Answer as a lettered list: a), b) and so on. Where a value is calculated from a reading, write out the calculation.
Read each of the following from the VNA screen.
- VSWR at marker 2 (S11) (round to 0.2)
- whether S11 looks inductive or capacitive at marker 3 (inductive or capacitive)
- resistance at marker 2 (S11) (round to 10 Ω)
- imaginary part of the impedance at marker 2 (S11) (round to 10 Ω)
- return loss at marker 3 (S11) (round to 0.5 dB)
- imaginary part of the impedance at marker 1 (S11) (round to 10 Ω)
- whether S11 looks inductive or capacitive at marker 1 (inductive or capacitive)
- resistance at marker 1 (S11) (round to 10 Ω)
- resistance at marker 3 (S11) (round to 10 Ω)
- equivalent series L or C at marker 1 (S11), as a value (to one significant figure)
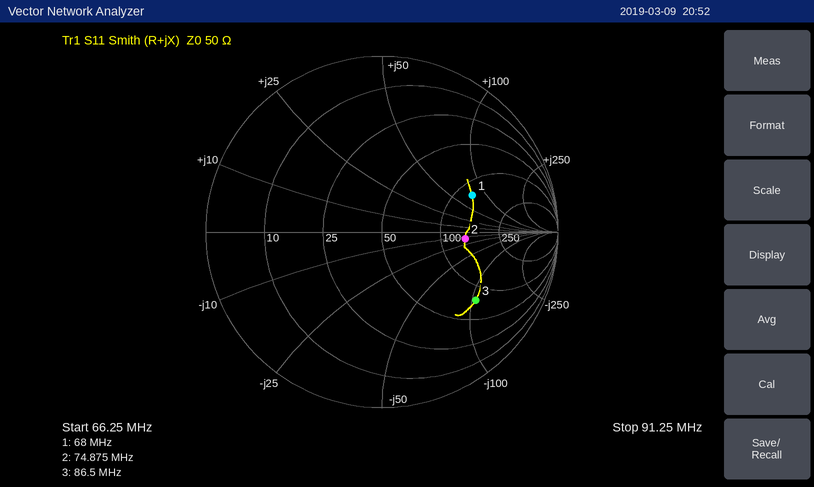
a) 2.8
b) capacitive
c) 140 Ω
d) -10 Ω
e) 3.5 dB
f) +70 Ω
g) inductive
h) 120 Ω
i) 80 Ω
j) L = 70 Ω/(2π × 68 MHz) ≈ 164 nH, so 200 nH to one significant figure
